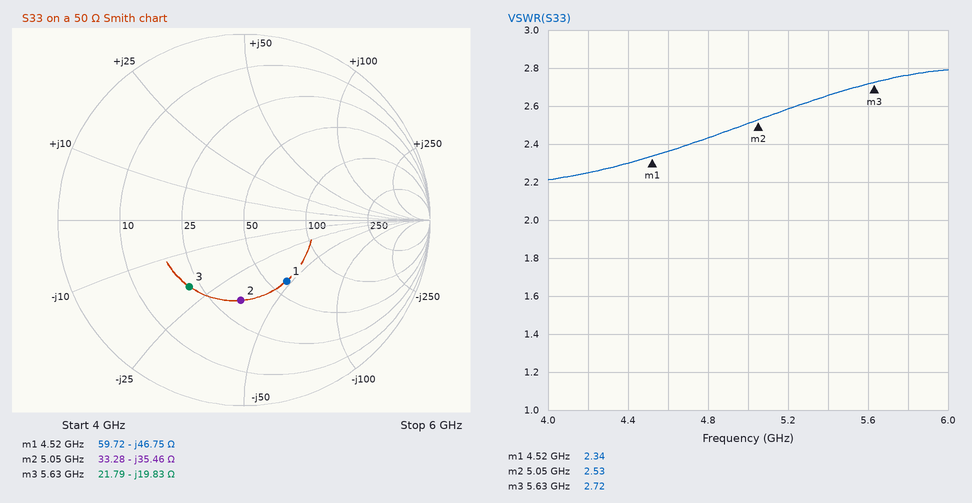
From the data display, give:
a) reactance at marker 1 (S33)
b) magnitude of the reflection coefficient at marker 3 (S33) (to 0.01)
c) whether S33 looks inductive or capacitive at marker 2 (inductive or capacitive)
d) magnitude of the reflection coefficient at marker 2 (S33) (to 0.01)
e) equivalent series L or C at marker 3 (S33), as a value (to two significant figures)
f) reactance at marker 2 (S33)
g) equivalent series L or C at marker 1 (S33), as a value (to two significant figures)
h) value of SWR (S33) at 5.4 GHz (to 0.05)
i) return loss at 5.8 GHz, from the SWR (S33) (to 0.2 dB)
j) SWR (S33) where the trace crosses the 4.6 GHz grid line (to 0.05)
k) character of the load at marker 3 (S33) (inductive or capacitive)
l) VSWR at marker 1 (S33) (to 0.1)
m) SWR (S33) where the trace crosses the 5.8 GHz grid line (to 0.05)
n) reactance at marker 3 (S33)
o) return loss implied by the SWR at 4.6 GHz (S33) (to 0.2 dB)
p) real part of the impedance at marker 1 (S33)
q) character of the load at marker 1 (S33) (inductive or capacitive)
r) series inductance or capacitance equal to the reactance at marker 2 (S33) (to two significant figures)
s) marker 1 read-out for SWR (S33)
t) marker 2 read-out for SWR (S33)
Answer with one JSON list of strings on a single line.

["-46.75 Ω", "0.46", "capacitive", "0.43", "1.4 pF", "-35.46 Ω", "750 fF", "2.65", "6.6 dB", "2.35", "capacitive", "2.3", "2.75", "-19.83 Ω", "7.8 dB", "59.72 Ω", "capacitive", "890 fF", "2.34", "2.53"]
